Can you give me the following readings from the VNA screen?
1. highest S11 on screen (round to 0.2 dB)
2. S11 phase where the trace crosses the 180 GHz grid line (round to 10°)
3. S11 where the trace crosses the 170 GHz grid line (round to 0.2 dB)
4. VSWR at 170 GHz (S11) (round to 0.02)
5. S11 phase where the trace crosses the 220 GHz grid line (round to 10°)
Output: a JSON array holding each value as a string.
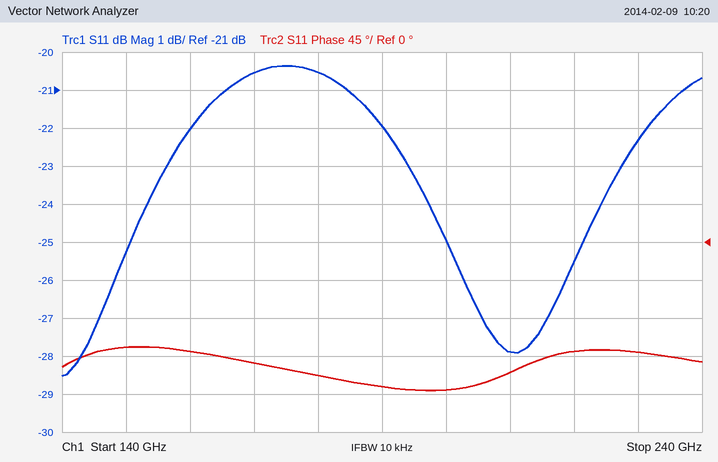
["-20.4 dB", "-160°", "-20.6 dB", "1.20", "-130°"]
